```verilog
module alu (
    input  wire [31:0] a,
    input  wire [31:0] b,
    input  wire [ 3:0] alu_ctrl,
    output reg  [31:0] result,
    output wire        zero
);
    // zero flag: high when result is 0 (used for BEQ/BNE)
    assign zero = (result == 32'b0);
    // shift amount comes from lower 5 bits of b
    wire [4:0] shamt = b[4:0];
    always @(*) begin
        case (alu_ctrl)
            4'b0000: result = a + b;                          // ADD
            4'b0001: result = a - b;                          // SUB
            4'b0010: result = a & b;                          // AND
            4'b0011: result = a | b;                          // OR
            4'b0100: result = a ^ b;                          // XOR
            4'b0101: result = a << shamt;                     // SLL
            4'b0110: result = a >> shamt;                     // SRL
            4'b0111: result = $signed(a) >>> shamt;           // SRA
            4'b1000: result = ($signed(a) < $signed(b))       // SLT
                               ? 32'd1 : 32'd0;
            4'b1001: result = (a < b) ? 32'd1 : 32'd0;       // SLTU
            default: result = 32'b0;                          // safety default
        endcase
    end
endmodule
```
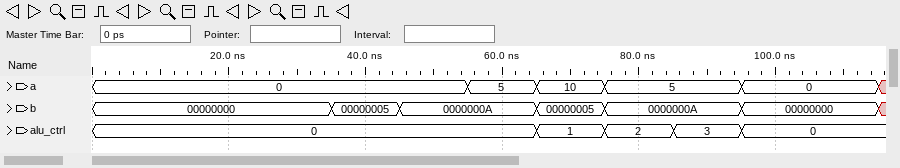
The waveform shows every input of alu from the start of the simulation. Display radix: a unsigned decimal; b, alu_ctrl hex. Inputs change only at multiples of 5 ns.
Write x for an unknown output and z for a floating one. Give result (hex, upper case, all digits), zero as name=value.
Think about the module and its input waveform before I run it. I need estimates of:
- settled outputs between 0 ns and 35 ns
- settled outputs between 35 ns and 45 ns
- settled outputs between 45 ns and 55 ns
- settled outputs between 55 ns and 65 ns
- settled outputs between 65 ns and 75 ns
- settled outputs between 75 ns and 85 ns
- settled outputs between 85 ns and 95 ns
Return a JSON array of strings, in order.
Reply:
["result=00000000, zero=1", "result=00000005, zero=0", "result=0000000A, zero=0", "result=0000000F, zero=0", "result=00000005, zero=0", "result=00000000, zero=1", "result=0000000F, zero=0"]
